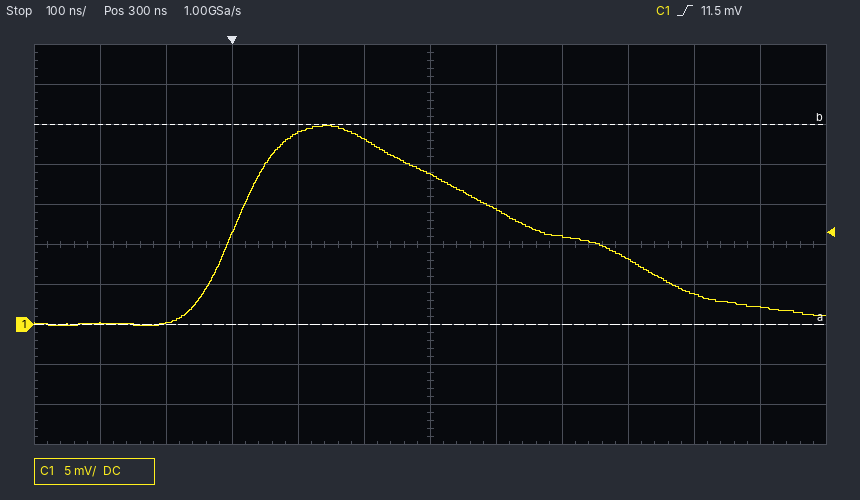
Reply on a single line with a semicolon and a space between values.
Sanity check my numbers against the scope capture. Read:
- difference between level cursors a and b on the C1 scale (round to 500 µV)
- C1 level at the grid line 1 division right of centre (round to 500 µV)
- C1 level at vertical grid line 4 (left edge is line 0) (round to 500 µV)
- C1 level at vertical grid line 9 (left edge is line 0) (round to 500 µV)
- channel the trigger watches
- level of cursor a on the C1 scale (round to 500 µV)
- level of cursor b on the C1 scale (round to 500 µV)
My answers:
25.0 mV; 14.5 mV; 24.0 mV; 8.0 mV; C1; 0.0 mV; 25.0 mV
